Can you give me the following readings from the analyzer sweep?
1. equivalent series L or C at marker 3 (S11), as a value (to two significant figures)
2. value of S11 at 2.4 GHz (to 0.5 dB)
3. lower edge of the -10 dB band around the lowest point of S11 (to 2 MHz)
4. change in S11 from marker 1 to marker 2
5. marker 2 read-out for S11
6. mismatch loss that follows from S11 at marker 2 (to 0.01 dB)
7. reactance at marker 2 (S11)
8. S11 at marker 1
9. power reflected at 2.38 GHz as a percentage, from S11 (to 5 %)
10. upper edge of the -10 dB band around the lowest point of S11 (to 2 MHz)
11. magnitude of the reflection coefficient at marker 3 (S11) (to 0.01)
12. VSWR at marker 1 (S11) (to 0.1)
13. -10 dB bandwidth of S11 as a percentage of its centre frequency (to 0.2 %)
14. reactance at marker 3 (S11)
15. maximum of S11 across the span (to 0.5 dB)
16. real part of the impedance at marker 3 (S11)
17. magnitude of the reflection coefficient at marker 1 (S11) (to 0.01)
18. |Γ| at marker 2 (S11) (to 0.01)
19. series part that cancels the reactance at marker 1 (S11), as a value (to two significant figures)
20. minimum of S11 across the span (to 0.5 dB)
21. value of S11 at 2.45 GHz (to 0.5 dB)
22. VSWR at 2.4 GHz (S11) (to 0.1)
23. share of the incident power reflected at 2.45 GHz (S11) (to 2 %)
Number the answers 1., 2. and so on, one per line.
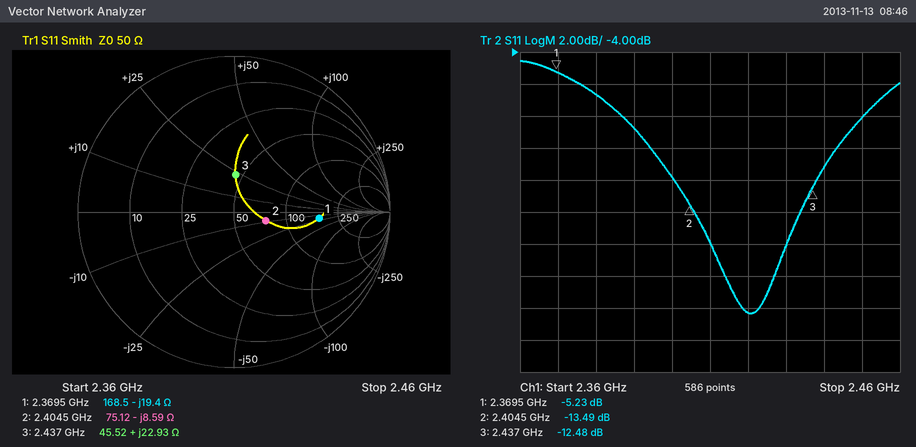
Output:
1. 1.5 nH
2. -12.0 dB
3. 2.394 GHz
4. -8.26 dB
5. -13.49 dB
6. 0.20 dB
7. -8.59 Ω
8. -5.23 dB
9. 20 %
10. 2.444 GHz
11. 0.24
12. 3.4
13. 2.0 %
14. +22.93 Ω
15. -4.5 dB
16. 45.52 Ω
17. 0.55
18. 0.21
19. 1.3 nH
20. -20.5 dB
21. -8.0 dB
22. 1.7
23. 16 %
